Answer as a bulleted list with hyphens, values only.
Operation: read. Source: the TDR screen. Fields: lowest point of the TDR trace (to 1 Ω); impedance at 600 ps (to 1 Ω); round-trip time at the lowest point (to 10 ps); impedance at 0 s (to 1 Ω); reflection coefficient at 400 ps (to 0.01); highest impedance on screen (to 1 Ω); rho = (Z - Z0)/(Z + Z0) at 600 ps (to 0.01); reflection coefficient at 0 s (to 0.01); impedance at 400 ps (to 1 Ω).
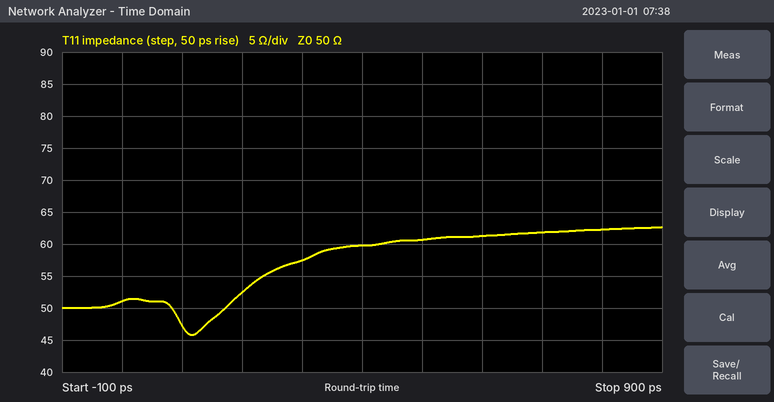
- 46 Ω
- 61 Ω
- 120 ps
- 51 Ω
- +0.09
- 63 Ω
- +0.10
- +0.01
- 60 Ω
